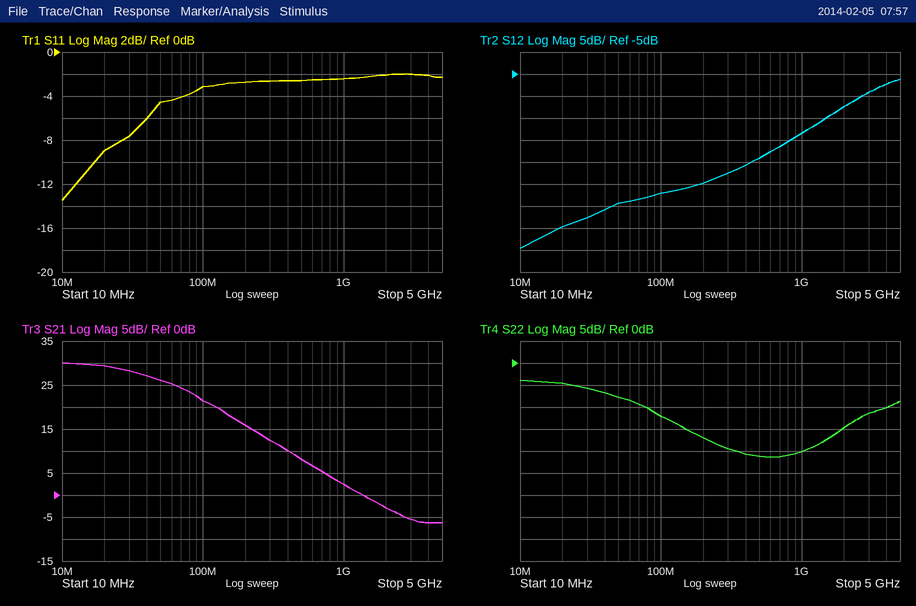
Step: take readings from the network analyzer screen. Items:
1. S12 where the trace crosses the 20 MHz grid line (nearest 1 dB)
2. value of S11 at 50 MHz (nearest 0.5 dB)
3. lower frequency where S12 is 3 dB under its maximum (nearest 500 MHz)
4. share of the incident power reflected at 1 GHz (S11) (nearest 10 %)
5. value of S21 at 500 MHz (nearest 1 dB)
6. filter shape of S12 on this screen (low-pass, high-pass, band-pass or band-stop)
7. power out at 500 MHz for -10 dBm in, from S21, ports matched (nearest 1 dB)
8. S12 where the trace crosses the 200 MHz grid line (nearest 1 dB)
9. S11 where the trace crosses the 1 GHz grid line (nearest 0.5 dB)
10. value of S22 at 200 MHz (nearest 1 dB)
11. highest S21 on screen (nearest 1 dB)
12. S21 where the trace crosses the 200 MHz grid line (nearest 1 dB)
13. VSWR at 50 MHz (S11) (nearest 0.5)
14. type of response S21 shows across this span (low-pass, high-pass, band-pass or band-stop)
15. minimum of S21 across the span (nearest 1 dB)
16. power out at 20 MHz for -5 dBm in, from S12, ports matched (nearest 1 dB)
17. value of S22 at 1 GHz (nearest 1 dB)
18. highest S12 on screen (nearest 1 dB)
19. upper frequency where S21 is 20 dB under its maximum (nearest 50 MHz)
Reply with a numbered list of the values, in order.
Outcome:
1. -40 dB
2. -4.5 dB
3. 3.0 GHz
4. 60 %
5. 8 dB
6. high-pass
7. -2 dBm
8. -30 dB
9. -2.5 dB
10. -17 dB
11. 30 dB
12. 16 dB
13. 4.0
14. low-pass
15. -6 dB
16. -45 dBm
17. -20 dB
18. -6 dB
19. 400 MHz
